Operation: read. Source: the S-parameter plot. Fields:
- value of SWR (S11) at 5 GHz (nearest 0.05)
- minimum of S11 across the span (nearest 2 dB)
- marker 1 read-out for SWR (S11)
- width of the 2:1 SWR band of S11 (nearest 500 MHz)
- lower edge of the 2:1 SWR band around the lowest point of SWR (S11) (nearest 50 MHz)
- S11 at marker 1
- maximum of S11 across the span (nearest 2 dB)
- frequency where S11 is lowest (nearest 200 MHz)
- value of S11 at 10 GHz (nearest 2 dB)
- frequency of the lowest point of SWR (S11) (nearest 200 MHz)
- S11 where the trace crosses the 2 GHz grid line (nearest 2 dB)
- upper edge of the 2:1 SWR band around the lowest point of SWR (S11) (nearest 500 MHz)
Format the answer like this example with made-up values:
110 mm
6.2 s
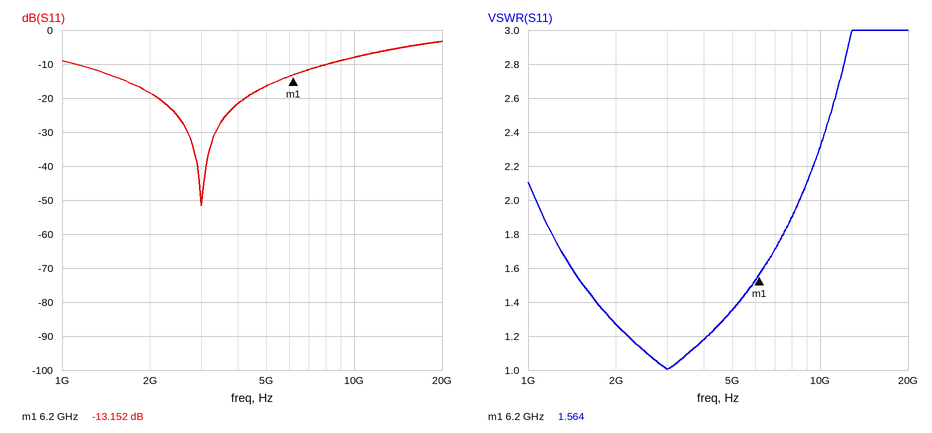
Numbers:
1.35
-52 dB
1.564
7.5 GHz
1.05 GHz
-13.152 dB
-4 dB
3.0 GHz
-8 dB
3.0 GHz
-18 dB
8.5 GHz
